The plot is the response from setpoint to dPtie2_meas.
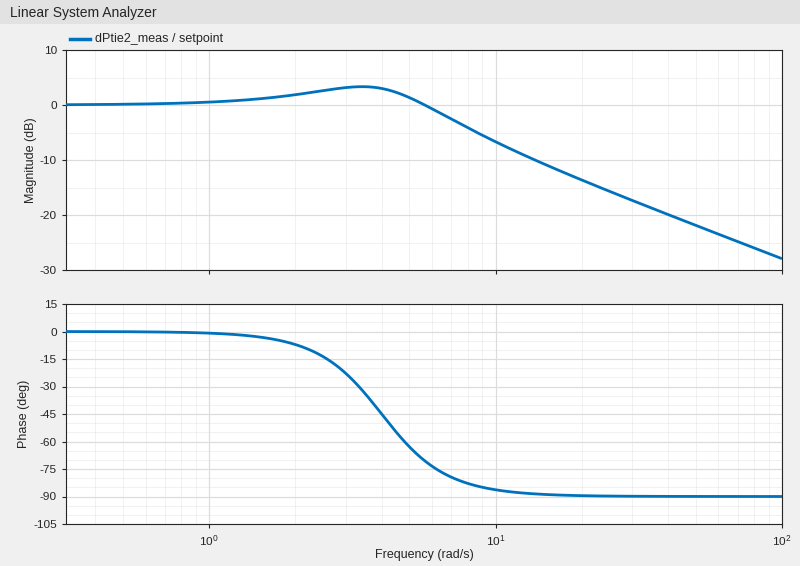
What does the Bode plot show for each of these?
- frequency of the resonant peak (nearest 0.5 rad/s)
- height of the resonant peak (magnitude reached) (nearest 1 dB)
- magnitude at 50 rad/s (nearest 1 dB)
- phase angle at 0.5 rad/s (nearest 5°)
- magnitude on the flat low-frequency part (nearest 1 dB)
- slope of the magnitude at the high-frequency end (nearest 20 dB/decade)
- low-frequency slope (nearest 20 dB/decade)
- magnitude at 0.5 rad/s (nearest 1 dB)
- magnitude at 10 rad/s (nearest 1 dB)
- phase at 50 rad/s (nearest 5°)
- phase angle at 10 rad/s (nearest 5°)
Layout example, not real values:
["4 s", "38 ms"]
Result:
["3.5 rad/s", "3 dB", "-22 dB", "0°", "0 dB", "-20 dB/decade", "0 dB/decade", "0 dB", "-7 dB", "-90°", "-85°"]
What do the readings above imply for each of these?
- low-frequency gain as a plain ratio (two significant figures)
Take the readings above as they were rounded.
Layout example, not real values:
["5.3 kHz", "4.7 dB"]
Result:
["1.0"]
